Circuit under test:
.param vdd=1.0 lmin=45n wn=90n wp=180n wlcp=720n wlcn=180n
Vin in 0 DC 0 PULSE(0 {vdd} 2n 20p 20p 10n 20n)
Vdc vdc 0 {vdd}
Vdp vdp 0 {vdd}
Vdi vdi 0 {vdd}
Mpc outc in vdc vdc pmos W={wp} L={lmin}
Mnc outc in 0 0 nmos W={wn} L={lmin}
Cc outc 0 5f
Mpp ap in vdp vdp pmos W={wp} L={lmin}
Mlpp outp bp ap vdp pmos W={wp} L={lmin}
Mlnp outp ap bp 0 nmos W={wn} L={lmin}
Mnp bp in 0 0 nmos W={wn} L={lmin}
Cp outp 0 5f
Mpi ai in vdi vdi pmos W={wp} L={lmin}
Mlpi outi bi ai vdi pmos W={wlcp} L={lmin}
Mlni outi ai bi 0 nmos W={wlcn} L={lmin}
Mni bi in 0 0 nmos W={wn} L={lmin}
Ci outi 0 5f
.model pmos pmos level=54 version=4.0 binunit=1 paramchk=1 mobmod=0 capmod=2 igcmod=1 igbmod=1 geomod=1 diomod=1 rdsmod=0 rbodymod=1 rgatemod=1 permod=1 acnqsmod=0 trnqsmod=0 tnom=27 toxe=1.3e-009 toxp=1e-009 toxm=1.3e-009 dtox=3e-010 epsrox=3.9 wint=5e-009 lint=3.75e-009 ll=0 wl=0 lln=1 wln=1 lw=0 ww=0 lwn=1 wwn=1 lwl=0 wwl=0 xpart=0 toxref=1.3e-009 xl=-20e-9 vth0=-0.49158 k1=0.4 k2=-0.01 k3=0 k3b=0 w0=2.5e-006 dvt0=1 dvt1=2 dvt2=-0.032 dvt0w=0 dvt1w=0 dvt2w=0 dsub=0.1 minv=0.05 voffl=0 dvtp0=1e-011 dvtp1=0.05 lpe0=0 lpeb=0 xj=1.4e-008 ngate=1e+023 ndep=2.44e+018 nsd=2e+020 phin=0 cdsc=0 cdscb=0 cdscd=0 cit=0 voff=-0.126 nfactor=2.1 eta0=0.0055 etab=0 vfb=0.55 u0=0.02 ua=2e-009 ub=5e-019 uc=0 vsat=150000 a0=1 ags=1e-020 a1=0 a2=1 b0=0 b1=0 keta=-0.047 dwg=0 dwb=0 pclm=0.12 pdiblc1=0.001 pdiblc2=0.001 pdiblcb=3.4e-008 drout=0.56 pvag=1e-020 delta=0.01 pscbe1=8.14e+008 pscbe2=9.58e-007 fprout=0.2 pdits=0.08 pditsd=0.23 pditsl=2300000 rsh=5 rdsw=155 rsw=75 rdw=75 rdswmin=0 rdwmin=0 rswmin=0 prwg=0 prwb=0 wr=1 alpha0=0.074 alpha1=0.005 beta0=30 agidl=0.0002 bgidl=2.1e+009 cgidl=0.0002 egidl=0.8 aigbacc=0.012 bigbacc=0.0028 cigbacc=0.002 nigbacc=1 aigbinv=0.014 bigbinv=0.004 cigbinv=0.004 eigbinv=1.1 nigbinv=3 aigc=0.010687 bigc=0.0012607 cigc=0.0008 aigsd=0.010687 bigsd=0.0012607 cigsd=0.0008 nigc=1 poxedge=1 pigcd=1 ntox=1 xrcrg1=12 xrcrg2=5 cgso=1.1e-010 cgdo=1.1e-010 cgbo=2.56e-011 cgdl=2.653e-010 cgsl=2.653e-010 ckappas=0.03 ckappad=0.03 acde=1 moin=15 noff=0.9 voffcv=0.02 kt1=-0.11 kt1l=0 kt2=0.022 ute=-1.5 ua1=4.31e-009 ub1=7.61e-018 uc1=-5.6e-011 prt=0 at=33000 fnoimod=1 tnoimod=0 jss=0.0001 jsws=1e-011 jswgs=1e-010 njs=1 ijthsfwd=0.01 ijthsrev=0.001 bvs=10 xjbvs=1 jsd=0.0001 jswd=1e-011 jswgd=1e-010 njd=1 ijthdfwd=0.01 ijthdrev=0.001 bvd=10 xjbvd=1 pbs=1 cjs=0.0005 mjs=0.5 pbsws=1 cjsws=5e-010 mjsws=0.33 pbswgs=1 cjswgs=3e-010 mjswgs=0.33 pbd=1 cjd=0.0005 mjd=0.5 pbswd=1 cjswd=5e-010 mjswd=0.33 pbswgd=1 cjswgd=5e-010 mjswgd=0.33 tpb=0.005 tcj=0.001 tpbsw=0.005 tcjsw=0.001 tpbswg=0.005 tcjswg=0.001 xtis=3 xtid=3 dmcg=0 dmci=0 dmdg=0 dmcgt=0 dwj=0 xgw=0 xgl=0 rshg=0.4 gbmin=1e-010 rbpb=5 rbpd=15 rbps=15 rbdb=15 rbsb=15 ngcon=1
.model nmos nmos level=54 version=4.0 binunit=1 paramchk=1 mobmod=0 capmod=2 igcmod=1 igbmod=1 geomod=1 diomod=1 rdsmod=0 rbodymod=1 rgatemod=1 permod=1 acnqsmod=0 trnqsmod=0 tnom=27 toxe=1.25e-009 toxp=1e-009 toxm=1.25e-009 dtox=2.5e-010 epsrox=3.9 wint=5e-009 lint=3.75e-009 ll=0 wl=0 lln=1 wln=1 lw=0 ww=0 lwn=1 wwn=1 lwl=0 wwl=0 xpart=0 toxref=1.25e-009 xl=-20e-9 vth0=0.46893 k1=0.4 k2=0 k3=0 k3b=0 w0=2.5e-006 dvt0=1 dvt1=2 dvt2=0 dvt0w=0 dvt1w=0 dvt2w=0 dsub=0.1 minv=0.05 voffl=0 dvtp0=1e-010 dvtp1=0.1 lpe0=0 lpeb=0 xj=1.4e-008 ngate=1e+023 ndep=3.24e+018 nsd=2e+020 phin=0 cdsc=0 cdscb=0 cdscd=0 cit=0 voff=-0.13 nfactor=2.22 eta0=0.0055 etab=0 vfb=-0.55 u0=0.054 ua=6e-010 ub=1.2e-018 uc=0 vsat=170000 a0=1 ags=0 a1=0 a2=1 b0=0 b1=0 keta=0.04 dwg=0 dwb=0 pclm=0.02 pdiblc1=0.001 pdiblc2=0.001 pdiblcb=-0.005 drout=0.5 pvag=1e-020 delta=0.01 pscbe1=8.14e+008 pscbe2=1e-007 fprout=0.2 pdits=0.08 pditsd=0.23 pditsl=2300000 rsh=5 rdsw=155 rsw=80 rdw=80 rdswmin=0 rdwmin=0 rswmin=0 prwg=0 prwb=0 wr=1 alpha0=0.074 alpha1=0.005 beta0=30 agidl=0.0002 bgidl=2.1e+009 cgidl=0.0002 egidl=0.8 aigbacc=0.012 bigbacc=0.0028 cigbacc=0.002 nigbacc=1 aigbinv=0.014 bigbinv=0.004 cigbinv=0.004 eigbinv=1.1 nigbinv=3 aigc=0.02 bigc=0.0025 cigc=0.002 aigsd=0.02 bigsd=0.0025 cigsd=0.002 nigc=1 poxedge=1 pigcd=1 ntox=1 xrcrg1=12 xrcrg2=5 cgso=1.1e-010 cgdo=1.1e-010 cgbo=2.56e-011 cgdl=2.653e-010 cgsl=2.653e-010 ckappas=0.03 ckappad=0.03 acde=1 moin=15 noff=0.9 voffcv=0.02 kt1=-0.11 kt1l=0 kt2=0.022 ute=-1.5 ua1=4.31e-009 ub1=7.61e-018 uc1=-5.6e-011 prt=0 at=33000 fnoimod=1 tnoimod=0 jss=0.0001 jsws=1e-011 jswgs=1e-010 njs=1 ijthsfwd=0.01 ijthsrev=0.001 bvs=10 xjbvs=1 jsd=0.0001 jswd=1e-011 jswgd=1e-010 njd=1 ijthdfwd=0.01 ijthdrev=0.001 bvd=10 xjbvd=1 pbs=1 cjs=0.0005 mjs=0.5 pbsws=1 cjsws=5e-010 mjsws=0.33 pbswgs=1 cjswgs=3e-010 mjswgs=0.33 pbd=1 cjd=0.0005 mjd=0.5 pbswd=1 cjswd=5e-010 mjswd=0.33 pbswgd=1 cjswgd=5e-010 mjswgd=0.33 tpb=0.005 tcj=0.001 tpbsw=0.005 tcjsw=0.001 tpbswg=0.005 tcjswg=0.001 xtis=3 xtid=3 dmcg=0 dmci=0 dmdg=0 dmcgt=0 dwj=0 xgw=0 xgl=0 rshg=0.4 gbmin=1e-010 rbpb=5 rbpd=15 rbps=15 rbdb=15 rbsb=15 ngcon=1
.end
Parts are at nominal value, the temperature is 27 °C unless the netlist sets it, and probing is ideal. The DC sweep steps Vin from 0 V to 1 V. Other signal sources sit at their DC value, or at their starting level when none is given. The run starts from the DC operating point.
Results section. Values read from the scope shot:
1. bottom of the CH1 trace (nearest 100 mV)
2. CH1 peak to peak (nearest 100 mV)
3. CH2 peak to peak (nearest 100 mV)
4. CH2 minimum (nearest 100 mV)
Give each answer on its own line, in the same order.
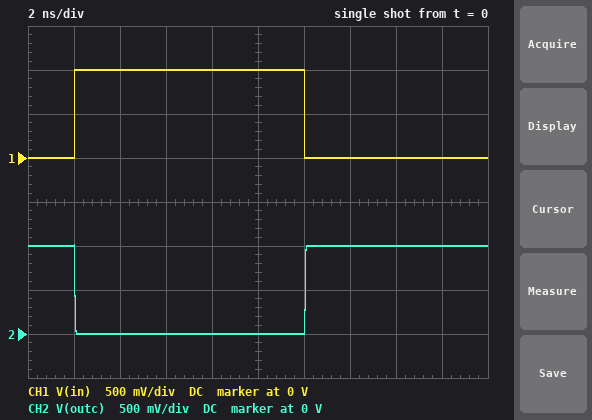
0 V
1.0 V
1.0 V
0 V
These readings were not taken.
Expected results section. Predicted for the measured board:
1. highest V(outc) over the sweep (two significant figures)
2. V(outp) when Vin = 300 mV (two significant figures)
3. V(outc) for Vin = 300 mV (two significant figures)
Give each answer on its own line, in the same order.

1.0 V
950 mV
990 mV
